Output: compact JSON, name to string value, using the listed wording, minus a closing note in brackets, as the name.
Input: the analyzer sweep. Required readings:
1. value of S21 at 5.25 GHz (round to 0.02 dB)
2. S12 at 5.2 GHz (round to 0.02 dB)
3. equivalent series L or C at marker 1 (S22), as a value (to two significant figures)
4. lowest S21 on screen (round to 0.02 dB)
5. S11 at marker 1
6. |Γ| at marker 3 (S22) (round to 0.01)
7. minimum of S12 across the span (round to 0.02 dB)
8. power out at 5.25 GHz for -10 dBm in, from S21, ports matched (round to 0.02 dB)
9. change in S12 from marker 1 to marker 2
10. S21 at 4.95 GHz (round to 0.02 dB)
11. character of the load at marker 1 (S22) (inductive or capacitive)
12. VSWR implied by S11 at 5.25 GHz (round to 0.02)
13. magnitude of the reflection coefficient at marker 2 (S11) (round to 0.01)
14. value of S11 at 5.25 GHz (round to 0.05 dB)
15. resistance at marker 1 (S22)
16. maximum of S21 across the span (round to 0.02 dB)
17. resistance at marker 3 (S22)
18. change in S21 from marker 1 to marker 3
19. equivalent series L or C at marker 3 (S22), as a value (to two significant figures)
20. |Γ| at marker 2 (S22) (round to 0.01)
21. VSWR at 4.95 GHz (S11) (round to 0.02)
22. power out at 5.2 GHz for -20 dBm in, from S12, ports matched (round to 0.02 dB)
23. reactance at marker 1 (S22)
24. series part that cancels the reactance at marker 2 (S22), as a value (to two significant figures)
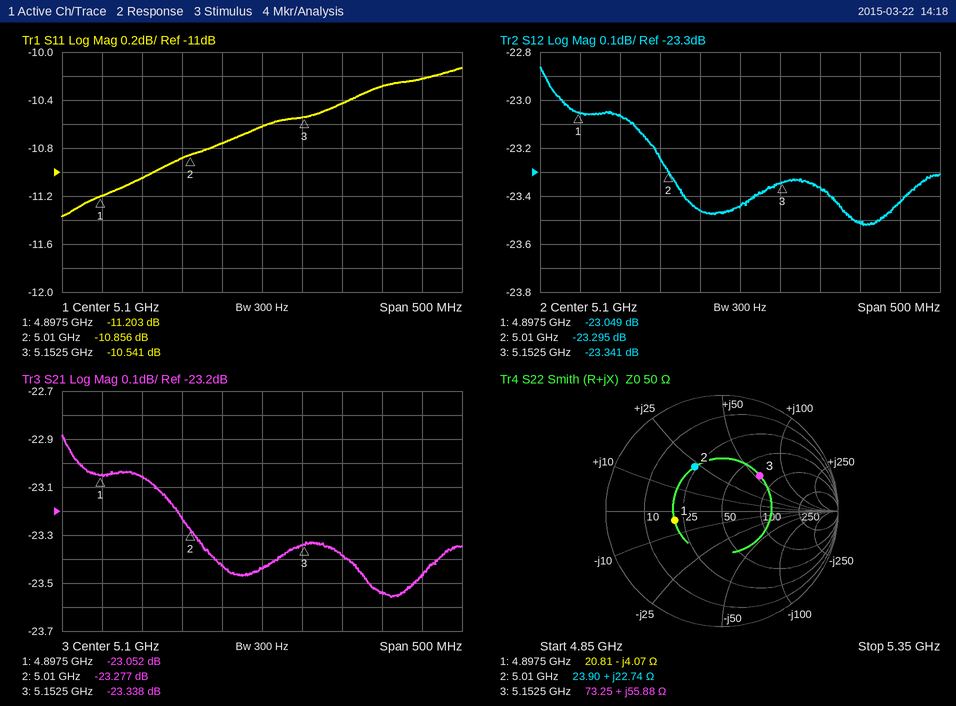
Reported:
{"value of S21 at 5.25 GHz": "-23.54 dB", "S12 at 5.2 GHz": "-23.36 dB", "equivalent series L or C at marker 1 (S22), as a value": "8.0 pF", "lowest S21 on screen": "-23.56 dB", "S11 at marker 1": "-11.203 dB", "|Γ| at marker 3 (S22)": "0.45", "minimum of S12 across the span": "-23.52 dB", "power out at 5.25 GHz for -10 dBm in, from S21, ports matched": "-33.54 dBm", "change in S12 from marker 1 to marker 2": "-0.246 dB", "S21 at 4.95 GHz": "-23.06 dB", "character of the load at marker 1 (S22)": "capacitive", "VSWR implied by S11 at 5.25 GHz": "1.88", "magnitude of the reflection coefficient at marker 2 (S11)": "0.29", "value of S11 at 5.25 GHz": "-10.30 dB", "resistance at marker 1": "20.81 Ω", "maximum of S21 across the span": "-22.88 dB", "resistance at marker 3": "73.25 Ω", "change in S21 from marker 1 to marker 3": "-0.286 dB", "equivalent series L or C at marker 3 (S22), as a value": "1.7 nH", "|Γ| at marker 2 (S22)": "0.45", "VSWR at 4.95 GHz (S11)": "1.78", "power out at 5.2 GHz for -20 dBm in, from S12, ports matched": "-43.36 dBm", "reactance at marker 1": "-4.07 Ω", "series part that cancels the reactance at marker 2 (S22), as a value": "1.4 pF"}
